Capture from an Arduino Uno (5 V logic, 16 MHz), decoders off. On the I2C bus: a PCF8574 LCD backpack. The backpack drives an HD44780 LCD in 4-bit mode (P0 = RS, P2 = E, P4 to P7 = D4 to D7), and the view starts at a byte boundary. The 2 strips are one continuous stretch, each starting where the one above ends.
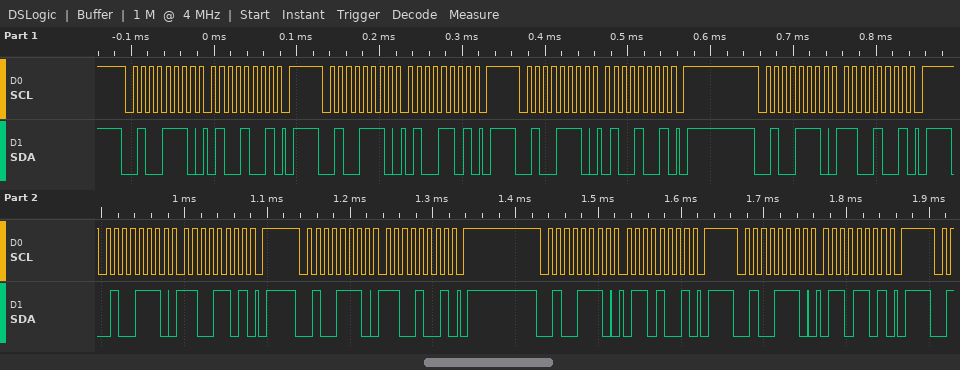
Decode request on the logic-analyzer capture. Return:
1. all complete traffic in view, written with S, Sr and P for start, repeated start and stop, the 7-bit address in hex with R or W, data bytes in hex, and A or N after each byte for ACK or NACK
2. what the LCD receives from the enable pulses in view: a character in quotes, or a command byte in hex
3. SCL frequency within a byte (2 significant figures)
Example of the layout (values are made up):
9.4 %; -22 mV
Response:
S 27W A 49 A P S 27W A 4D A P S 27W A 49 A P S 27W A C9 A P S 27W A CD A P S 27W A C9 A P S 27W A 69 A P S 27W A 6D A P; 'L'; 100 kHz
